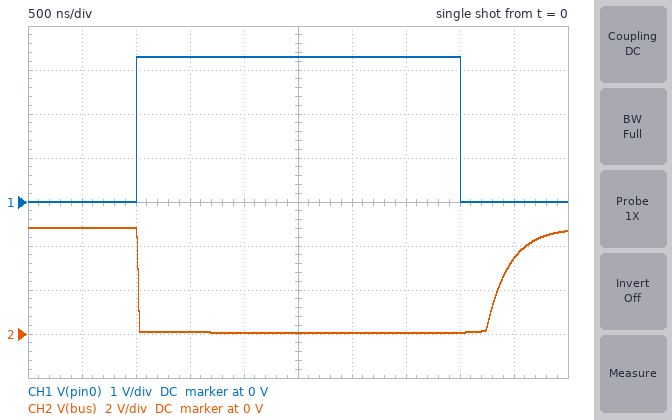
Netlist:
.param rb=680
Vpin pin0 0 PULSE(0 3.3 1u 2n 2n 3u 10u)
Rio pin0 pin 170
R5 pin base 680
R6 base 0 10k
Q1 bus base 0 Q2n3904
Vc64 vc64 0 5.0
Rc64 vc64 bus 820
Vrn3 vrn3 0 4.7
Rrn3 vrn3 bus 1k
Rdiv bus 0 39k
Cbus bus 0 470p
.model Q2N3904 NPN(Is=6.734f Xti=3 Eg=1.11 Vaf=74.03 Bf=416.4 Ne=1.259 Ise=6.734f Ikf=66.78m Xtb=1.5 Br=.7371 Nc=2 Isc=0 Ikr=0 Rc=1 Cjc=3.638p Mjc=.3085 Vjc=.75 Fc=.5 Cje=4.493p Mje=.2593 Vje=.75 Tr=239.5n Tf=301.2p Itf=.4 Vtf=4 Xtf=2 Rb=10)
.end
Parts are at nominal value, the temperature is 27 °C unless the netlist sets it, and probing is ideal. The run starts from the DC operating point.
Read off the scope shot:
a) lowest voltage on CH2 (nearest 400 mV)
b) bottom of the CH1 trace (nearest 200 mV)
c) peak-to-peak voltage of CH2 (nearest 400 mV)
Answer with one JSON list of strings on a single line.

["0 V", "0 V", "4.8 V"]
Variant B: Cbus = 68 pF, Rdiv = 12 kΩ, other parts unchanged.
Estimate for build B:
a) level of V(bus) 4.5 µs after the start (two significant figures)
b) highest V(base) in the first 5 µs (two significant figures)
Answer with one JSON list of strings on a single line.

["4.7 V", "810 mV"]
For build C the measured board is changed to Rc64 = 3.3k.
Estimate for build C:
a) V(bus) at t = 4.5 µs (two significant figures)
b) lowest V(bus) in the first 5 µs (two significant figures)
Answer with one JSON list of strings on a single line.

["2.4 V", "42 mV"]
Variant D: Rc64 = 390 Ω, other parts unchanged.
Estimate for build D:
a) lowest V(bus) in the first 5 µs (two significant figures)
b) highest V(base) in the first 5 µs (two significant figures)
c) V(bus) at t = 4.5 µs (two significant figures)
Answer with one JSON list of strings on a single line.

["81 mV", "840 mV", "4.3 V"]
